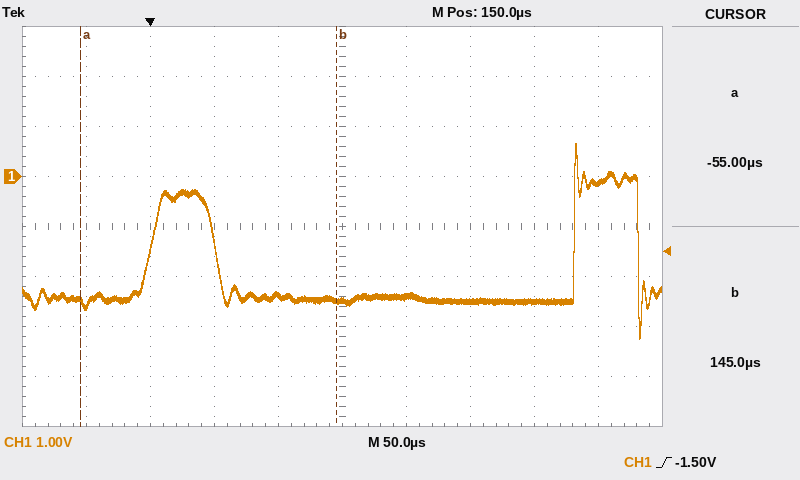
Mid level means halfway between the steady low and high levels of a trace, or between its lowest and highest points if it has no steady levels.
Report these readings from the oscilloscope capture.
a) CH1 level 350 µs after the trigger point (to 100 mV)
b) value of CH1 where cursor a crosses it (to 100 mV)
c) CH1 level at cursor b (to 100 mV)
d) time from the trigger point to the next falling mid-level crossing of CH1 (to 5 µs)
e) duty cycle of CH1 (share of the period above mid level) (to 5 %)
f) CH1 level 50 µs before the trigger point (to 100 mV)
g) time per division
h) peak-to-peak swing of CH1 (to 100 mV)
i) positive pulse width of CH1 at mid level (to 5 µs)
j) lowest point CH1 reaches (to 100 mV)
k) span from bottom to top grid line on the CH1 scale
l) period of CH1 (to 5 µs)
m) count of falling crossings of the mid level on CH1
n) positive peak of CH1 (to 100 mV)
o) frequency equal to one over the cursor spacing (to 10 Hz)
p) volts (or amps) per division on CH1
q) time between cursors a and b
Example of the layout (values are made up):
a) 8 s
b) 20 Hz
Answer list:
a) -100 mV
b) -2.5 V
c) -2.5 V
d) 50 µs
e) 15 %
f) -2.6 V
g) 50 µs
h) 3.9 V
i) 50 µs
j) -3.2 V
k) 8 V
l) 330 µs
m) 2
n) 700 mV
o) 5.00 kHz
p) 1 V
q) 200 µs
